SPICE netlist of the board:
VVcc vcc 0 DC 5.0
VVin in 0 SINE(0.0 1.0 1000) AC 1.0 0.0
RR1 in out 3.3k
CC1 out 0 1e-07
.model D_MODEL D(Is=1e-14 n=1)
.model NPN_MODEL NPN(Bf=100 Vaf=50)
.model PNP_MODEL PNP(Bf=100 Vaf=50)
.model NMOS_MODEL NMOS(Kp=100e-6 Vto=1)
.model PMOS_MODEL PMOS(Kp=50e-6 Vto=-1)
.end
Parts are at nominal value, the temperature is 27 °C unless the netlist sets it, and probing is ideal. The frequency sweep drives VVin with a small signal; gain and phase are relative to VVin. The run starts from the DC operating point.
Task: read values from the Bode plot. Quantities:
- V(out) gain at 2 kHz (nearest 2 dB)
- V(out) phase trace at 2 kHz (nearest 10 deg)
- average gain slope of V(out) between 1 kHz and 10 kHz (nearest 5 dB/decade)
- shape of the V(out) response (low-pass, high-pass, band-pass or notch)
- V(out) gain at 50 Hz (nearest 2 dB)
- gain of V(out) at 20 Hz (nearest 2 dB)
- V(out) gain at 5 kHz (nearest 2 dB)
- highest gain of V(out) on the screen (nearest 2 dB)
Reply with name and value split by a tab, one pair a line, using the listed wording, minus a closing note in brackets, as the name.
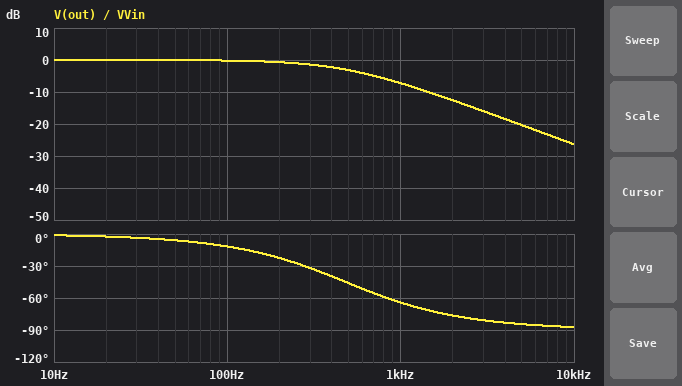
V(out) gain at 2 kHz	-12 dB
V(out) phase trace at 2 kHz	-80 deg
average gain slope of V(out) between 1 kHz and 10 kHz	-20 dB/decade
shape of the V(out) response	low-pass
V(out) gain at 50 Hz	0 dB
gain of V(out) at 20 Hz	0 dB
V(out) gain at 5 kHz	-20 dB
highest gain of V(out) on the screen	0 dB
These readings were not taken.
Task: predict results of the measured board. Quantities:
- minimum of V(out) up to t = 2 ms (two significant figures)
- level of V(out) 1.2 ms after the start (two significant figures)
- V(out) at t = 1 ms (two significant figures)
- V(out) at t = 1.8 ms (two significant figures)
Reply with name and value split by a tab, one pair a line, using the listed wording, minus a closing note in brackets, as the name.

minimum of V(out) up to t = 2 ms	-430 mV
level of V(out) 1.2 ms after the start	69 mV
V(out) at t = 1 ms	-370 mV
V(out) at t = 1.8 ms	-300 mV
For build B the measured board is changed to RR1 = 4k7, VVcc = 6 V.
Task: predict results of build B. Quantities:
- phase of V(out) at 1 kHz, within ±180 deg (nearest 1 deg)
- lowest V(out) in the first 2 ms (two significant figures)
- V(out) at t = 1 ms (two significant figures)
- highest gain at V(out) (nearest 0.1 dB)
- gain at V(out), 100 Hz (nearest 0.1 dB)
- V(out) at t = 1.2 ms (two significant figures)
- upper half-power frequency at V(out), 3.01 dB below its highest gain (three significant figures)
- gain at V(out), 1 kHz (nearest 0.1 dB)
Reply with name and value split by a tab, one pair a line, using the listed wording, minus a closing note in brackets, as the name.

phase of V(out) at 1 kHz, within ±180 deg	-71 deg
lowest V(out) in the first 2 ms	-320 mV
V(out) at t = 1 ms	-270 mV
highest gain at V(out)	0 dB
gain at V(out), 100 Hz	-0.4 dB
V(out) at t = 1.2 ms	28 mV
upper half-power frequency at V(out), 3.01 dB below its highest gain	339 Hz
gain at V(out), 1 kHz	-9.9 dB
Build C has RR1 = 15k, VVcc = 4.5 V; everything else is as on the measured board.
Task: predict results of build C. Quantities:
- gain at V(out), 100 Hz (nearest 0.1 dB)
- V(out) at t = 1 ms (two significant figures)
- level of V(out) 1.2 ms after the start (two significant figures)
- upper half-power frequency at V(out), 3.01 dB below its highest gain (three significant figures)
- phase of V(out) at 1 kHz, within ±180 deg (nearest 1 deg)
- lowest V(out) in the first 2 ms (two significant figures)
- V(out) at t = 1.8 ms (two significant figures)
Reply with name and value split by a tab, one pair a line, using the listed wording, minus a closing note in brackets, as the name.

gain at V(out), 100 Hz	-2.8 dB
V(out) at t = 1 ms	-51 mV
level of V(out) 1.2 ms after the start	25 mV
upper half-power frequency at V(out), 3.01 dB below its highest gain	106 Hz
phase of V(out) at 1 kHz, within ±180 deg	-84 deg
lowest V(out) in the first 2 ms	-78 mV
V(out) at t = 1.8 ms	-11 mV
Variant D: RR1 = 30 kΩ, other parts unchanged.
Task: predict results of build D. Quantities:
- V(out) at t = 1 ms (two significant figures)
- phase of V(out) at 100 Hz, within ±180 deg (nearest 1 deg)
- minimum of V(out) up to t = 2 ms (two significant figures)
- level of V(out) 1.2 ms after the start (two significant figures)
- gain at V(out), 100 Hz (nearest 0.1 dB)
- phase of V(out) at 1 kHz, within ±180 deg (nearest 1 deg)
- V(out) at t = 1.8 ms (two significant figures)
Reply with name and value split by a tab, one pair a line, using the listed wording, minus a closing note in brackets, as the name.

V(out) at t = 1 ms	-15 mV
phase of V(out) at 100 Hz, within ±180 deg	-62 deg
minimum of V(out) up to t = 2 ms	-26 mV
level of V(out) 1.2 ms after the start	22 mV
gain at V(out), 100 Hz	-6.6 dB
phase of V(out) at 1 kHz, within ±180 deg	-87 deg
V(out) at t = 1.8 ms	10 mV
